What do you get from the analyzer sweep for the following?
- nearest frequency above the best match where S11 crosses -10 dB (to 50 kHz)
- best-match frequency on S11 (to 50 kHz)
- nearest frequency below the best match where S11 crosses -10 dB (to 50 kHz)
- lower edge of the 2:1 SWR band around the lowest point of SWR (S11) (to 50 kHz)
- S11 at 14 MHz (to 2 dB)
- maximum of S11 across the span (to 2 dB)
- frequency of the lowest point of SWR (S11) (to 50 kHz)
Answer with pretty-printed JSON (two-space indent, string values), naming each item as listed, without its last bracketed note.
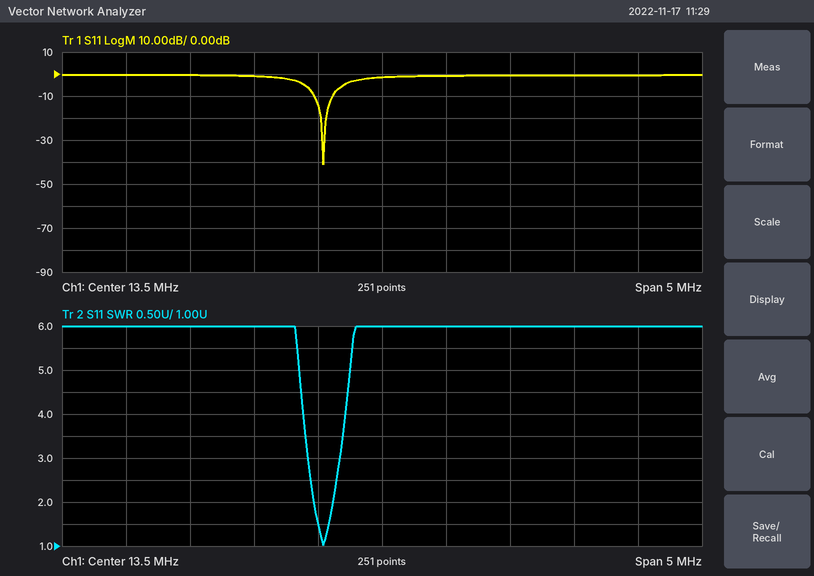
{
  "nearest frequency above the best match where S11 crosses -10 dB": "13.10 MHz",
  "best-match frequency on S11": "13.05 MHz",
  "nearest frequency below the best match where S11 crosses -10 dB": "12.95 MHz",
  "lower edge of the 2:1 SWR band around the lowest point of SWR (S11)": "12.95 MHz",
  "S11 at 14 MHz": "0 dB",
  "maximum of S11 across the span": "0 dB",
  "frequency of the lowest point of SWR (S11)": "13.05 MHz"
}
